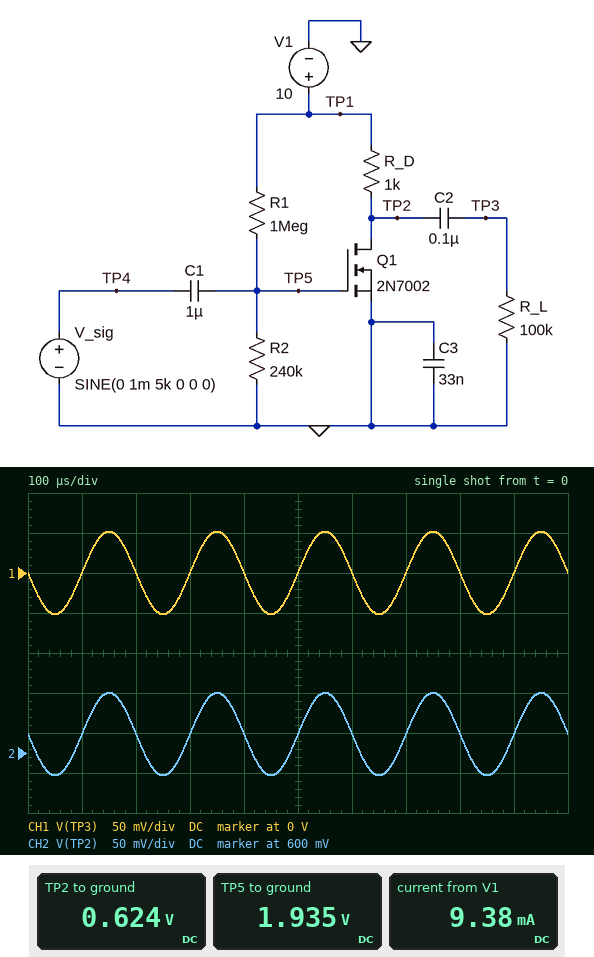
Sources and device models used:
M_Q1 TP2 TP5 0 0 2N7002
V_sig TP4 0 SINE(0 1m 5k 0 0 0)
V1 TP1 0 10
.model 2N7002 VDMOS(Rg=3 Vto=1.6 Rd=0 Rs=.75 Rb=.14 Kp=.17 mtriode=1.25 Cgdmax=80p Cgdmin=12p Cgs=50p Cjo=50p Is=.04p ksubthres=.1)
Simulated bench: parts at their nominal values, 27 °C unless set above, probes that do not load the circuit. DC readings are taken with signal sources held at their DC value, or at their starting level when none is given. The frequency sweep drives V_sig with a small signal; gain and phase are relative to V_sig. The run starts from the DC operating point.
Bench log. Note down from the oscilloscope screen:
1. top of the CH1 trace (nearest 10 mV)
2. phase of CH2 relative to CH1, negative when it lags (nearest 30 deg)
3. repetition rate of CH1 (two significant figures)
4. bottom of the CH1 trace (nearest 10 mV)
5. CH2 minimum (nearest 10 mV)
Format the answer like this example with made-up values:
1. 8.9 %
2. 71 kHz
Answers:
1. 50 mV
2. 0 deg
3. 5.0 kHz
4. -50 mV
5. 570 mV
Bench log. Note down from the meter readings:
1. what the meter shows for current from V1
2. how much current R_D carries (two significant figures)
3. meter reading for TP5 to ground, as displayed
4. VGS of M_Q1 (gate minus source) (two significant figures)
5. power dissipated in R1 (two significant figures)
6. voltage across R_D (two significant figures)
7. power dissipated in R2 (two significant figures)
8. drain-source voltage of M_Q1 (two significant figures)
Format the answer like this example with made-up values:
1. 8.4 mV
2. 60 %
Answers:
1. 9.38 mA
2. 9.4 mA
3. 1.935 V
4. 1.9 V
5. 65 µW
6. 9.4 V
7. 16 µW
8. 620 mV
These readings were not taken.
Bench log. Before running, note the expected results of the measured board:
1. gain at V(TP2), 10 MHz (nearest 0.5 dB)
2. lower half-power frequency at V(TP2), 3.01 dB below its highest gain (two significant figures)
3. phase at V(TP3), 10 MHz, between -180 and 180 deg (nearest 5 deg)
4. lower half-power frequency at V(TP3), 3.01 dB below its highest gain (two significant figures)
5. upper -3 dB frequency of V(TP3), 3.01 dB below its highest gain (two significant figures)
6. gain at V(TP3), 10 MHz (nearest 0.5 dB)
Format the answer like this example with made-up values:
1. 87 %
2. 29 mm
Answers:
1. 16.5 dB
2. 810 mHz
3. 90 deg
4. 16 Hz
5. 1.3 MHz
6. 16.5 dB
